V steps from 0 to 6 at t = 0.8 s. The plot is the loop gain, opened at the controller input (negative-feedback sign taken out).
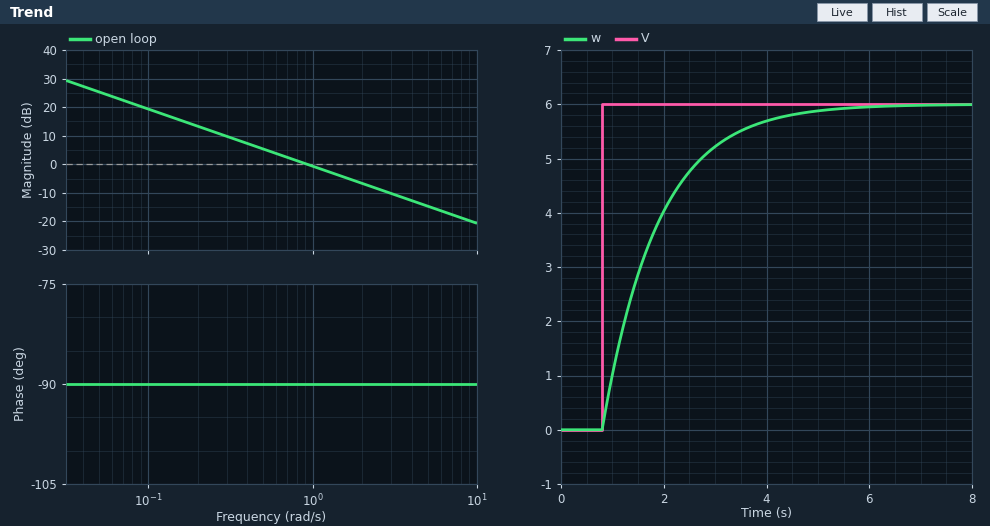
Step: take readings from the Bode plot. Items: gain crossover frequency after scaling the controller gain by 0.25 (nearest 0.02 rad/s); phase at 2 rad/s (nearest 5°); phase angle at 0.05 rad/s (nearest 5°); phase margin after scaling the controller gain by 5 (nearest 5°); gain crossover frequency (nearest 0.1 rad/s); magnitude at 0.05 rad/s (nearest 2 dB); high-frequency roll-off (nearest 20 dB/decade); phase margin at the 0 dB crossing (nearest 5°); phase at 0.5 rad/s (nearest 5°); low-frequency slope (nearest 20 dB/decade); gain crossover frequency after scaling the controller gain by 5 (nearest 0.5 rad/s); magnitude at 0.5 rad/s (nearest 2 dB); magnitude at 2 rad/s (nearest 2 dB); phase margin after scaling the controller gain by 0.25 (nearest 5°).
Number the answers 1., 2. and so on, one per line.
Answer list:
1. 0.24 rad/s
2. -90°
3. -90°
4. 90°
5. 0.9 rad/s
6. 26 dB
7. -20 dB/decade
8. 90°
9. -90°
10. -20 dB/decade
11. 4.5 rad/s
12. 6 dB
13. -6 dB
14. 90°
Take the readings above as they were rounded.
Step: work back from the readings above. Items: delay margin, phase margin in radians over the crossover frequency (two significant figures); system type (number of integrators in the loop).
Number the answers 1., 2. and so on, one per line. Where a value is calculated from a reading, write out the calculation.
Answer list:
1. 90 × π / 180 / 0.9 = 1.7 s
2. 1
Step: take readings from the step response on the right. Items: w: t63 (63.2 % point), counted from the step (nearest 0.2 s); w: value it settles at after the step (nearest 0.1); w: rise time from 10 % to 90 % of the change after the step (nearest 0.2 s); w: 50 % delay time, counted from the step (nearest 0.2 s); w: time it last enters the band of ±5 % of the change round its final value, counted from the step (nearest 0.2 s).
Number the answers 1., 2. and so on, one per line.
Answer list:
1. 1.0 s
2. 6.0
3. 2.4 s
4. 0.8 s
5. 3.2 s
